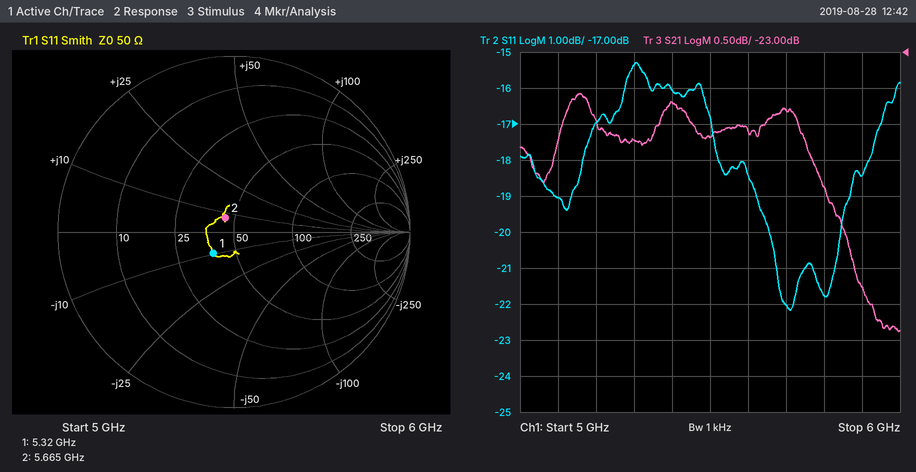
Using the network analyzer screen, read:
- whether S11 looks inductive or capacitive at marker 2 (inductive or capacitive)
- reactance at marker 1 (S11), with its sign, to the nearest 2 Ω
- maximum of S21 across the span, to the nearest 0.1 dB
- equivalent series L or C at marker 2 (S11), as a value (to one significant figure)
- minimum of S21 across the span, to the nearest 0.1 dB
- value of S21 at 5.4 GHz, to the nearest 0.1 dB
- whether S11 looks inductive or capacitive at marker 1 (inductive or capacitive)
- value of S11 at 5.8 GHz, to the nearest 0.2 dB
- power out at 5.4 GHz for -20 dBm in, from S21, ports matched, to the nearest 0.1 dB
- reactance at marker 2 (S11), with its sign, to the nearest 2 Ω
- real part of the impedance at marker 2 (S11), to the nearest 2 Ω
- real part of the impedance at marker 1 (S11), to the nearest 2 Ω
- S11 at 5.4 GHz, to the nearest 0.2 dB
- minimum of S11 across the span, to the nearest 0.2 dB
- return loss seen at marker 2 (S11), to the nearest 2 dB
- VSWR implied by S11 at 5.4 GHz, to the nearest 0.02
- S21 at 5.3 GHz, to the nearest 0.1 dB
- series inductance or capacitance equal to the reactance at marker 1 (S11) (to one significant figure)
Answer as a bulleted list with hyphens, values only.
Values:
- inductive
- -10 Ω
- -23.6 dB
- 200 pH
- -26.9 dB
- -23.7 dB
- capacitive
- -21.8 dB
- -43.7 dBm
- +8 Ω
- 44 Ω
- 38 Ω
- -16.0 dB
- -22.2 dB
- 20 dB
- 1.38
- -24.2 dB
- 3 pF
